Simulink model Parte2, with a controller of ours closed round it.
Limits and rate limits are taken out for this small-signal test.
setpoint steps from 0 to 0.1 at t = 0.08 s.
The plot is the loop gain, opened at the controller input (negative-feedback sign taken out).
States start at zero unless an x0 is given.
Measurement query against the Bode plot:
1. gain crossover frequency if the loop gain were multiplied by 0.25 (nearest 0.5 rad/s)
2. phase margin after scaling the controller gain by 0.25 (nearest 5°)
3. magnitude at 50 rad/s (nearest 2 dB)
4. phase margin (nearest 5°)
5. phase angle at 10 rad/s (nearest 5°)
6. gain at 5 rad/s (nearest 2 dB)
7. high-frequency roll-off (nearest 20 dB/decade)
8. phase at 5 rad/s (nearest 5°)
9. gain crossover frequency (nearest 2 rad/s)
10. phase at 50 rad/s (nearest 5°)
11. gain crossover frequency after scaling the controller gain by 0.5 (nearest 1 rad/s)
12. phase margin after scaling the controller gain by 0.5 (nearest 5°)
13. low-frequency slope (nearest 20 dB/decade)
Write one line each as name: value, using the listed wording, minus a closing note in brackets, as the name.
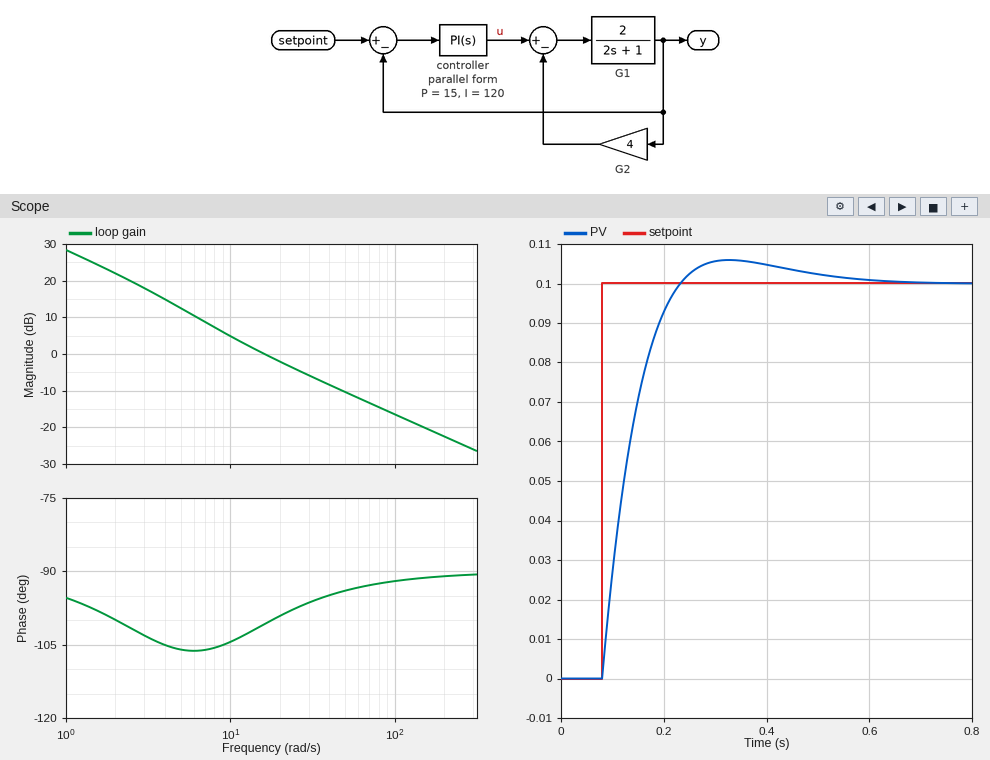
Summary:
gain crossover frequency if the loop gain were multiplied by 0.25: 5.0 rad/s
phase margin after scaling the controller gain by 0.25: 75°
magnitude at 50 rad/s: -10 dB
phase margin: 80°
phase angle at 10 rad/s: -105°
gain at 5 rad/s: 12 dB
high-frequency roll-off: -20 dB/decade
phase at 5 rad/s: -105°
gain crossover frequency: 16 rad/s
phase at 50 rad/s: -95°
gain crossover frequency after scaling the controller gain by 0.5: 9 rad/s
phase margin after scaling the controller gain by 0.5: 75°
low-frequency slope: -20 dB/decade
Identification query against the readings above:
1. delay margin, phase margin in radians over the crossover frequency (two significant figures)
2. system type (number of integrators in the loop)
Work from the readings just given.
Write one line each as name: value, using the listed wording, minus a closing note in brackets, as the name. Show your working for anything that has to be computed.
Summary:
delay margin, phase margin in radians over the crossover frequency: 80 × π / 180 / 16 = 0.087 s
system type: 1
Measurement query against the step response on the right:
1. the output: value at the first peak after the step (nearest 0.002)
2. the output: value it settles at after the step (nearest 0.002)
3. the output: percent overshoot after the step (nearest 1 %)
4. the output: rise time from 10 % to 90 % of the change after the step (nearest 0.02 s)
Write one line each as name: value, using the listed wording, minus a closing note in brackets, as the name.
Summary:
the output: value at the first peak after the step: 0.106
the output: value it settles at after the step: 0.100
the output: percent overshoot after the step: 6 %
the output: rise time from 10 % to 90 % of the change after the step: 0.10 s
